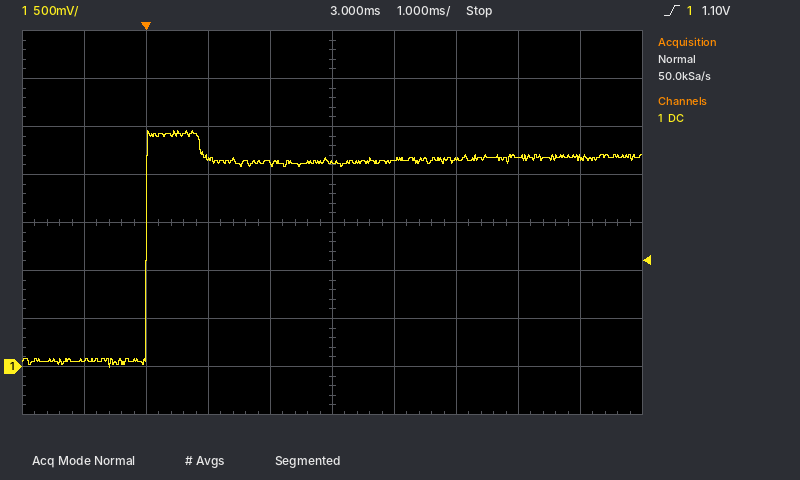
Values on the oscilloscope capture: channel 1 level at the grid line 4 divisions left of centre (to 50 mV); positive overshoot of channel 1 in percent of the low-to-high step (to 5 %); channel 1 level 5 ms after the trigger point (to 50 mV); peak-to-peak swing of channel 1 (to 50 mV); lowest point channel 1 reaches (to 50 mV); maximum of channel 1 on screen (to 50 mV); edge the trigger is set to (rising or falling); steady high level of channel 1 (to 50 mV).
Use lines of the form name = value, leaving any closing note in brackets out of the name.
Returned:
channel 1 level at the grid line 4 divisions left of centre = 50 mV
positive overshoot of channel 1 in percent of the low-to-high step = 15 %
channel 1 level 5 ms after the trigger point = 2.15 V
peak-to-peak swing of channel 1 = 2.45 V
lowest point channel 1 reaches = 0 mV
maximum of channel 1 on screen = 2.45 V
edge the trigger is set to = rising
steady high level of channel 1 = 2.15 V
